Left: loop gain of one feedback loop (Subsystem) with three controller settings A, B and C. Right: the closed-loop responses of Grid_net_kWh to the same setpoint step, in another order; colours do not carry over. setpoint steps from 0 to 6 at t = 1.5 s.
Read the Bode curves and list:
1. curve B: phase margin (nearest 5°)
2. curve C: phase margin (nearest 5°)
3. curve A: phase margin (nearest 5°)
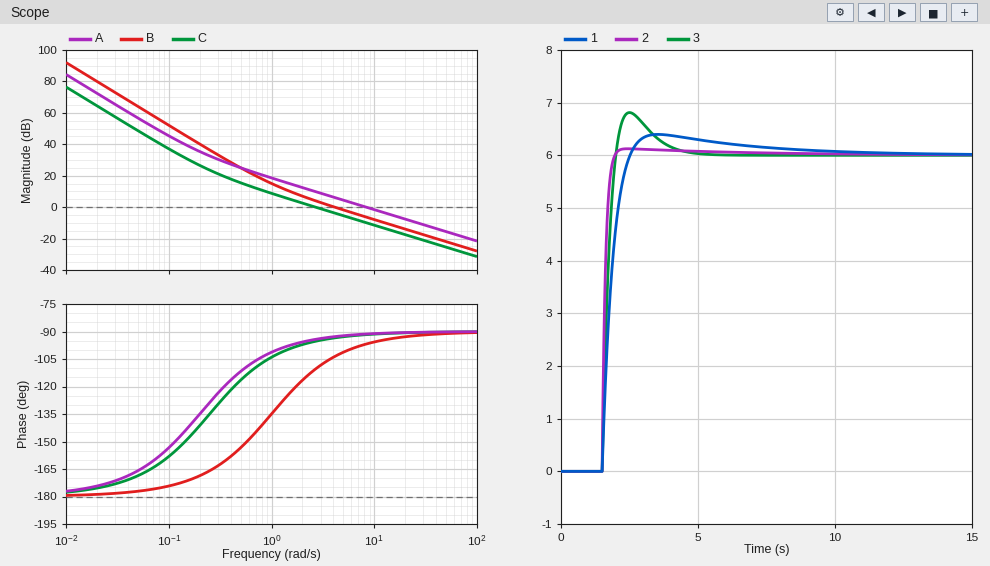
75°
85°
90°
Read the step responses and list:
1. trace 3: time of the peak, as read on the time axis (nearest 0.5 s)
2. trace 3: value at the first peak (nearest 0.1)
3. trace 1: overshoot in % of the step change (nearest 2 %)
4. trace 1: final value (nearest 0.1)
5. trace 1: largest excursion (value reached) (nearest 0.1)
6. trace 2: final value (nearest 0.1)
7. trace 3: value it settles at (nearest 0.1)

2.5 s
6.8
6 %
6.0
6.4
6.0
6.0
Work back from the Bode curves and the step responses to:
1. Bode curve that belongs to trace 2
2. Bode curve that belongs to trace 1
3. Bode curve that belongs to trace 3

A
C
B
